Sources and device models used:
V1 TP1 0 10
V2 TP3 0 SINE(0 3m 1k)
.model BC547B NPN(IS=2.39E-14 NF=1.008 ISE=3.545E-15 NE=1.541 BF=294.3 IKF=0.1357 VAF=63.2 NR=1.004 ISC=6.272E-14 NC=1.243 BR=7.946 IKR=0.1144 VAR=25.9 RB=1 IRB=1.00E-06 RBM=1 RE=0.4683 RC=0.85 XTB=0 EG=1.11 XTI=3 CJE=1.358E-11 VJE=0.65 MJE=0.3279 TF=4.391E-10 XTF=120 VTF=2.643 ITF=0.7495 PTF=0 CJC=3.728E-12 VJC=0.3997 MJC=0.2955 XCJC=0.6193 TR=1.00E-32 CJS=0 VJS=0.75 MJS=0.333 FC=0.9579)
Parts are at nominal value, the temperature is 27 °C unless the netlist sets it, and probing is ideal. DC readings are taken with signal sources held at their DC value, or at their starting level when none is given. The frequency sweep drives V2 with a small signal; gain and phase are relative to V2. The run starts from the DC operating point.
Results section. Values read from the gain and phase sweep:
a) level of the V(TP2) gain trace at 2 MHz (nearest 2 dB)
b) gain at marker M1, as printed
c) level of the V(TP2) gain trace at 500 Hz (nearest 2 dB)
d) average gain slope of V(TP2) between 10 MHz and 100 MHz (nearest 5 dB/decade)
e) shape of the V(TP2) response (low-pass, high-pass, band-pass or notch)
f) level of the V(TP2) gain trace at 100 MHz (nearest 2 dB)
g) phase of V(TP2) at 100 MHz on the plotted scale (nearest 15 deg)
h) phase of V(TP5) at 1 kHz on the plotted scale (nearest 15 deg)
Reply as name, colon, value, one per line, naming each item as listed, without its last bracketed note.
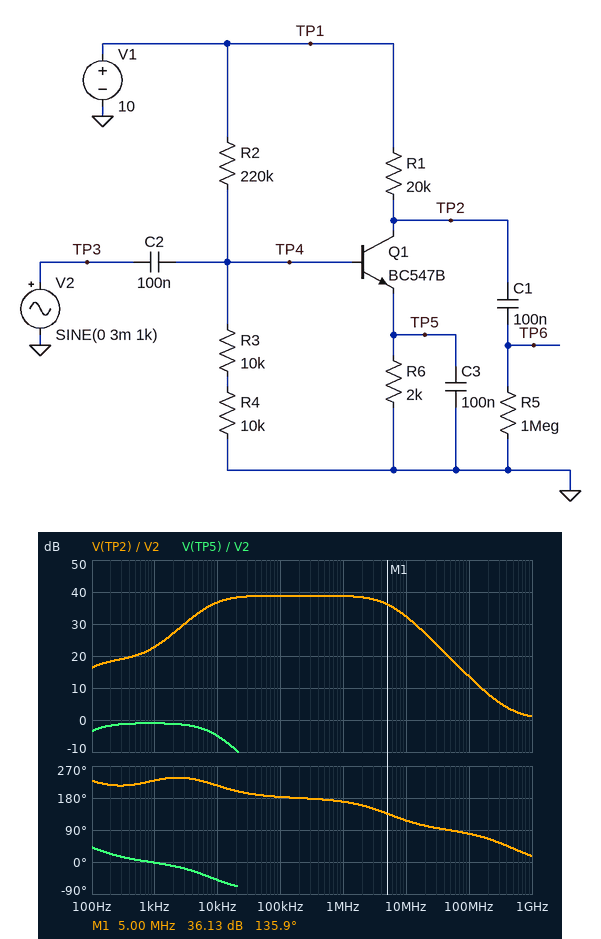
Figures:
level of the V(TP2) gain trace at 2 MHz: 38 dB
gain at marker M1, as printed: 36.13 dB
level of the V(TP2) gain trace at 500 Hz: 20 dB
average gain slope of V(TP2) between 10 MHz and 100 MHz: -20 dB/decade
shape of the V(TP2) response: band-pass
level of the V(TP2) gain trace at 100 MHz: 14 dB
phase of V(TP2) at 100 MHz on the plotted scale: 75 deg
phase of V(TP5) at 1 kHz on the plotted scale: 0 deg
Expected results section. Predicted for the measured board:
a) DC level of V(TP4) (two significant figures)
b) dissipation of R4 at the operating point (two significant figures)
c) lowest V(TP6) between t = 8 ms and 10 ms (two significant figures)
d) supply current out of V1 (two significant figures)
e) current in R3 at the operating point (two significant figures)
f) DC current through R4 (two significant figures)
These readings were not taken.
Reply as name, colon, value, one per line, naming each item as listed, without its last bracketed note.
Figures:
DC level of V(TP4): 830 mV
dissipation of R4 at the operating point: 17 µW
lowest V(TP6) between t = 8 ms and 10 ms: -42 mV
supply current out of V1: 160 µA
current in R3 at the operating point: 41 µA
DC current through R4: 41 µA
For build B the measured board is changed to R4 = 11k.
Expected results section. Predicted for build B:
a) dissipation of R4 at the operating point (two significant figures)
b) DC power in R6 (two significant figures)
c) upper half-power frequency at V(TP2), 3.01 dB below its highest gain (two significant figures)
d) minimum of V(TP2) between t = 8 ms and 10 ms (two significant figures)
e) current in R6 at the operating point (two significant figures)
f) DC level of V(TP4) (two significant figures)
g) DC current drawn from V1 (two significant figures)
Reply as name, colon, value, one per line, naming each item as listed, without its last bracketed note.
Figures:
dissipation of R4 at the operating point: 19 µW
DC power in R6: 39 µW
upper half-power frequency at V(TP2), 3.01 dB below its highest gain: 5.2 MHz
minimum of V(TP2) between t = 8 ms and 10 ms: 7.2 V
current in R6 at the operating point: 140 µA
DC level of V(TP4): 860 mV
DC current drawn from V1: 180 µA
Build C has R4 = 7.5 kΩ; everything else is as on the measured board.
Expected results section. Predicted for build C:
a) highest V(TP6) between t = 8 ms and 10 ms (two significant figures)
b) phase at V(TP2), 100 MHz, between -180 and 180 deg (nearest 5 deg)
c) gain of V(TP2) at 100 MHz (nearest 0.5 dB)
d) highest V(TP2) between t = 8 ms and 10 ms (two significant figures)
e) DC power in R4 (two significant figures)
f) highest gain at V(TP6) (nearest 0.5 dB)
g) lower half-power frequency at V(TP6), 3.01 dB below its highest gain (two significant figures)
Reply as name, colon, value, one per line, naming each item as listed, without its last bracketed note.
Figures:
highest V(TP6) between t = 8 ms and 10 ms: 39 mV
phase at V(TP2), 100 MHz, between -180 and 180 deg: 75 deg
gain of V(TP2) at 100 MHz: 10.5 dB
highest V(TP2) between t = 8 ms and 10 ms: 8.4 V
DC power in R4: 13 µW
highest gain at V(TP6): 35.5 dB
lower half-power frequency at V(TP6), 3.01 dB below its highest gain: 5.5 kHz
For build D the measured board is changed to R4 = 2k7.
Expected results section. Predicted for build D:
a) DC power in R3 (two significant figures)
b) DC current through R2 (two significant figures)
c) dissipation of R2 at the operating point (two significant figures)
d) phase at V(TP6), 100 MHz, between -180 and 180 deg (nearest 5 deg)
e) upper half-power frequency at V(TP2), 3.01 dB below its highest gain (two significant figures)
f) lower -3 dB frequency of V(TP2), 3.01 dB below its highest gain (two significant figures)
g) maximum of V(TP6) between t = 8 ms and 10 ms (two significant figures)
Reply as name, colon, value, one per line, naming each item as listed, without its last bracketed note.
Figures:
DC power in R3: 18 µW
DC current through R2: 43 µA
dissipation of R2 at the operating point: 410 µW
phase at V(TP6), 100 MHz, between -180 and 180 deg: 30 deg
upper half-power frequency at V(TP2), 3.01 dB below its highest gain: 5.7 MHz
lower -3 dB frequency of V(TP2), 3.01 dB below its highest gain: 1.1 kHz
maximum of V(TP6) between t = 8 ms and 10 ms: 19 mV
